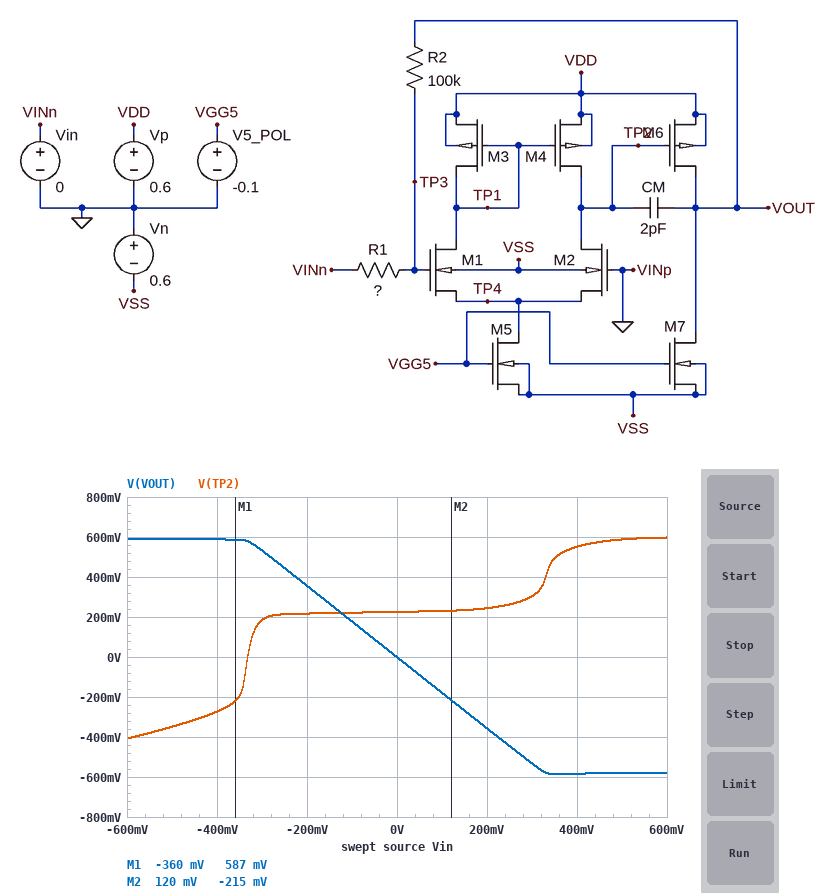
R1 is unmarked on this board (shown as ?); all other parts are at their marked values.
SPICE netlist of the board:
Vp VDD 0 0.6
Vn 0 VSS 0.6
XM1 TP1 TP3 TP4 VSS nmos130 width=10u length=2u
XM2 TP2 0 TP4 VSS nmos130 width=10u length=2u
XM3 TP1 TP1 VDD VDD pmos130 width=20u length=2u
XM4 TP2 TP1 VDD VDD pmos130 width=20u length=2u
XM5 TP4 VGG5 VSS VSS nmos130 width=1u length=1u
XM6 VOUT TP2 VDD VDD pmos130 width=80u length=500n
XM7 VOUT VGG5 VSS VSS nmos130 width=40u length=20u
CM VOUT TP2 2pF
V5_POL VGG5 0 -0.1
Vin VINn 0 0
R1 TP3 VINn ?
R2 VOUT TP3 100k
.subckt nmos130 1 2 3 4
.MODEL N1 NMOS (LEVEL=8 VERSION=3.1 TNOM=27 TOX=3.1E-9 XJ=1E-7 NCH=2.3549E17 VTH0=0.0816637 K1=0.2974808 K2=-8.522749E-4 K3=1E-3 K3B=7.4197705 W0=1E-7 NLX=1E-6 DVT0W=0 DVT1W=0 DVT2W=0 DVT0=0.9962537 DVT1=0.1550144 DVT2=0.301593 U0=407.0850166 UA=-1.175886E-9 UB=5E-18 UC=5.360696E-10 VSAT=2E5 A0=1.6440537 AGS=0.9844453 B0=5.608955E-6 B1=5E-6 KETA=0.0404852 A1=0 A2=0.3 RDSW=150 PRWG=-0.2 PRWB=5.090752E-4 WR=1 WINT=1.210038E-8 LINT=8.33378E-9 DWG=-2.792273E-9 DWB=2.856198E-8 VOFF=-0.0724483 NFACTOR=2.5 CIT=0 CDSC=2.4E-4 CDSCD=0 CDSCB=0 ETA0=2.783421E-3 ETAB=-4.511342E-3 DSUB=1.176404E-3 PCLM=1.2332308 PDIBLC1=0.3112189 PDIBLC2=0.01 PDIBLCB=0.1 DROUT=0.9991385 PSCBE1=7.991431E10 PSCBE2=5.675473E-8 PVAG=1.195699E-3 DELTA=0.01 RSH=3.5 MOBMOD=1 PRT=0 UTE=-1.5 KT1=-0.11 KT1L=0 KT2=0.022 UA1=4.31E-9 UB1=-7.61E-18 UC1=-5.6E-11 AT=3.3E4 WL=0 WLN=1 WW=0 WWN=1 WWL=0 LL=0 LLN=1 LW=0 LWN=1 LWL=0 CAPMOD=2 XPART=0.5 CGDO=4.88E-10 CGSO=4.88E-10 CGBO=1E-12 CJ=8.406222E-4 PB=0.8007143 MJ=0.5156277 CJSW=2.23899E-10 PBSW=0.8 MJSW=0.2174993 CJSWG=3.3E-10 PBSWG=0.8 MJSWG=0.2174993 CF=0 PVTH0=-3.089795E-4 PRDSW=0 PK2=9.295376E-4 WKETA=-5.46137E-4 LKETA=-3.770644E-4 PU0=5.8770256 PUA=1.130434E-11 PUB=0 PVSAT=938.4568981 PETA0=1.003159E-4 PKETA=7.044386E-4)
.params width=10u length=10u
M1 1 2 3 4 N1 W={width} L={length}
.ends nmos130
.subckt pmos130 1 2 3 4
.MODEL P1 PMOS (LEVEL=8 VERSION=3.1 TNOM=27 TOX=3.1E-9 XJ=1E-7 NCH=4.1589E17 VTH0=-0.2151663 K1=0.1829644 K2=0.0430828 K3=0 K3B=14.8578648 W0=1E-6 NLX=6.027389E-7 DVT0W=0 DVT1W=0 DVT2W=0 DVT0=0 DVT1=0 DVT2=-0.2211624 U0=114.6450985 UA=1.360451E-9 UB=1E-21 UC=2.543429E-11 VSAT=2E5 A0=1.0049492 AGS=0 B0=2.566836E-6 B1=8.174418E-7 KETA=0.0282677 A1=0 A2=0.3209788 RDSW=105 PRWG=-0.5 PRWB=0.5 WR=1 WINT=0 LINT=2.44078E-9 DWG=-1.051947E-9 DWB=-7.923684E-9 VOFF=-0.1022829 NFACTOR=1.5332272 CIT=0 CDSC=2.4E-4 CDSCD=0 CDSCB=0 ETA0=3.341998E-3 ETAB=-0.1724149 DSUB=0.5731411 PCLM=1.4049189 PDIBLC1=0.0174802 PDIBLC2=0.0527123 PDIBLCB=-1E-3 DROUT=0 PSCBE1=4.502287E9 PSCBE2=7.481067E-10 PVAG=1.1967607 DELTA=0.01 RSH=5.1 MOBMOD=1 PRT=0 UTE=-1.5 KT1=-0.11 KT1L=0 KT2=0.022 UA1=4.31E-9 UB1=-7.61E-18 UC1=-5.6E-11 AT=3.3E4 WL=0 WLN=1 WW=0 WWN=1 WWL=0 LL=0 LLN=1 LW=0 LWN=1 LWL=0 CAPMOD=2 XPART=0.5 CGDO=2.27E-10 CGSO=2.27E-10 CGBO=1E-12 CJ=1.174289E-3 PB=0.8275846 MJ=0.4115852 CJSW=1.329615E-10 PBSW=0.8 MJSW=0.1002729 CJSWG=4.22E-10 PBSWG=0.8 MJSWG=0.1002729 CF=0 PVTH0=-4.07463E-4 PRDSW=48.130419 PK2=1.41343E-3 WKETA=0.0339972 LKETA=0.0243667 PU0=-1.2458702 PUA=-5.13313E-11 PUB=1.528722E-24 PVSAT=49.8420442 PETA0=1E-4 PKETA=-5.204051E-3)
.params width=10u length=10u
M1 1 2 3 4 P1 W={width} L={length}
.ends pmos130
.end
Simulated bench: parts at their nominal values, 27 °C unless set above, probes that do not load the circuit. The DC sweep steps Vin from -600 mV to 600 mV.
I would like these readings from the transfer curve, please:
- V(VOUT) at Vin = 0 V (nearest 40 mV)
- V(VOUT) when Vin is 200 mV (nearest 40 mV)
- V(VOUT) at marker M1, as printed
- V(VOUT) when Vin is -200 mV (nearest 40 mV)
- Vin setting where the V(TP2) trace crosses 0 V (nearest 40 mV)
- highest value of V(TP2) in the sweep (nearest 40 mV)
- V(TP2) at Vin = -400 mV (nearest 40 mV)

0 V
-360 mV
587 mV
360 mV
-320 mV
600 mV
-280 mV
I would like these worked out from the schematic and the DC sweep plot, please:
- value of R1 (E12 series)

56 kΩ
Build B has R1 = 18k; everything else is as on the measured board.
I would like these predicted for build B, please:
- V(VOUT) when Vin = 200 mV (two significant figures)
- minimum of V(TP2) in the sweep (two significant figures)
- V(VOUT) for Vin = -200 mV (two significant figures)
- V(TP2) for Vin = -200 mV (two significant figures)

-580 mV
-570 mV
590 mV
-320 mV
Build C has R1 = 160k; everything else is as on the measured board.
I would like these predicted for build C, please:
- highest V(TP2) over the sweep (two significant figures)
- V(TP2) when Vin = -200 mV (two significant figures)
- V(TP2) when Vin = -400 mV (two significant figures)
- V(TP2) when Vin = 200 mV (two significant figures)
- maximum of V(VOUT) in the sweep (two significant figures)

250 mV
220 mV
220 mV
230 mV
370 mV
